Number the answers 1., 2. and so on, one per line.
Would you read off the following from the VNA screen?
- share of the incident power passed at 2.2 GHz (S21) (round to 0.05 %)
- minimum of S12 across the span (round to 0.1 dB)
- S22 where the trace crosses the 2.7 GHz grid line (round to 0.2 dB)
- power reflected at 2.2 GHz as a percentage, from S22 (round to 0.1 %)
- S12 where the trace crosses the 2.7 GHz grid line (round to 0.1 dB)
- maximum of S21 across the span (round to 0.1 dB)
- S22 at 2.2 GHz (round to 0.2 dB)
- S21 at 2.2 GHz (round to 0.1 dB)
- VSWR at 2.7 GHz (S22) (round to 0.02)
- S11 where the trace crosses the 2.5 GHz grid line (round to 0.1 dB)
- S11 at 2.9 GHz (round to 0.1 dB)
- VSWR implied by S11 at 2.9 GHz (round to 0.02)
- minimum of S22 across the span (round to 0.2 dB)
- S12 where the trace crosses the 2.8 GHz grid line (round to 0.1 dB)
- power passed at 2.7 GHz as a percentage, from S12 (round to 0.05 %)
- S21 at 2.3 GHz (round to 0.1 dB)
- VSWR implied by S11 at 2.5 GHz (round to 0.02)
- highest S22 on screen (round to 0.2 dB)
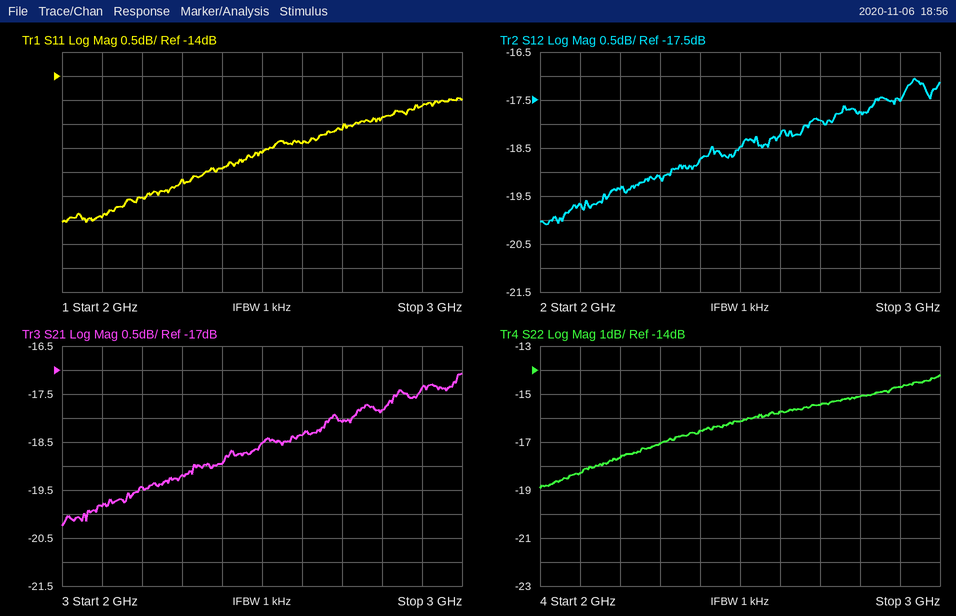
1. 1.15 %
2. -20.1 dB
3. -15.4 dB
4. 1.7 %
5. -17.9 dB
6. -17.1 dB
7. -17.6 dB
8. -19.4 dB
9. 1.40
10. -15.6 dB
11. -14.6 dB
12. 1.46
13. -19.0 dB
14. -17.7 dB
15. 1.60 %
16. -19.2 dB
17. 1.40
18. -14.2 dB
